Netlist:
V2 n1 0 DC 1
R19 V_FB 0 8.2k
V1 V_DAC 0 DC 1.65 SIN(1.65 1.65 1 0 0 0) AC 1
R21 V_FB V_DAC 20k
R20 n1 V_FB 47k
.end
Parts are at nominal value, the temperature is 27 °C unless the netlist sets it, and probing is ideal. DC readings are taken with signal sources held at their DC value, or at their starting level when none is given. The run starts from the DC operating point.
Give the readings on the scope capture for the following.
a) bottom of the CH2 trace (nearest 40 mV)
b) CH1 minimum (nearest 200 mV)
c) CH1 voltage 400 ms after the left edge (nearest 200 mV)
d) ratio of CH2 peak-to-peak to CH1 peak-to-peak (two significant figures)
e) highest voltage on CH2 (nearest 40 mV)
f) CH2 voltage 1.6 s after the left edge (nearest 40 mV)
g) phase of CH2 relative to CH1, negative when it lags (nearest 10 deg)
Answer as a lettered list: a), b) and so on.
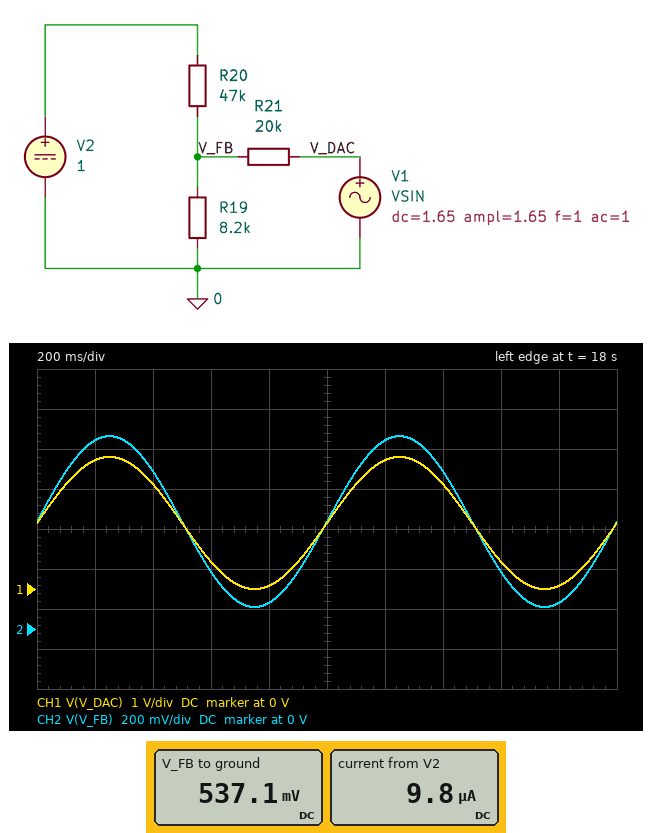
a) 120 mV
b) 0 V
c) 2.6 V
d) 0.26
e) 960 mV
f) 280 mV
g) 0 deg
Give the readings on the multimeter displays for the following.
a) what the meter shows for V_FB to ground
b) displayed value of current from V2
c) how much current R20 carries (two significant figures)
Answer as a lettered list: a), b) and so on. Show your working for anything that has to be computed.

a) 537.1 mV
b) 9.8 µA
c) (1 V - 537.1 mV) / 47 kΩ = 9.8 µA
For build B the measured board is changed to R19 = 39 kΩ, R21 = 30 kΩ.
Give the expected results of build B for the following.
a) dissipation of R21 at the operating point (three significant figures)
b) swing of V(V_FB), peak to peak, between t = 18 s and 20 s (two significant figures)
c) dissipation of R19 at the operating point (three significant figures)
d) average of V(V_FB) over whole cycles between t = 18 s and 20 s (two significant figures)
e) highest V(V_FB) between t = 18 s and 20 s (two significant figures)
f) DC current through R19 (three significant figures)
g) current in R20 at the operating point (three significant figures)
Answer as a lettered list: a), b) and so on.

a) 16.3 µW
b) 1.4 V
c) 23.2 µW
d) 950 mV
e) 1.6 V
f) 24.4 µA
g) 1.05 µA
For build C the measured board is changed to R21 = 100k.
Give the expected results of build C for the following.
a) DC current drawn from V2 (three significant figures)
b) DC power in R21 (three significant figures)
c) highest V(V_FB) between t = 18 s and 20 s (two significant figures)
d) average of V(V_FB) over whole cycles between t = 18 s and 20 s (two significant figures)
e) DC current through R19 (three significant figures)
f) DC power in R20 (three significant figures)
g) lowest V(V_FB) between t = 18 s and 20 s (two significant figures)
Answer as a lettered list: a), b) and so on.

a) 16.0 µA
b) 19.7 µW
c) 350 mV
d) 250 mV
e) 30.1 µA
f) 12.1 µW
g) 140 mV
